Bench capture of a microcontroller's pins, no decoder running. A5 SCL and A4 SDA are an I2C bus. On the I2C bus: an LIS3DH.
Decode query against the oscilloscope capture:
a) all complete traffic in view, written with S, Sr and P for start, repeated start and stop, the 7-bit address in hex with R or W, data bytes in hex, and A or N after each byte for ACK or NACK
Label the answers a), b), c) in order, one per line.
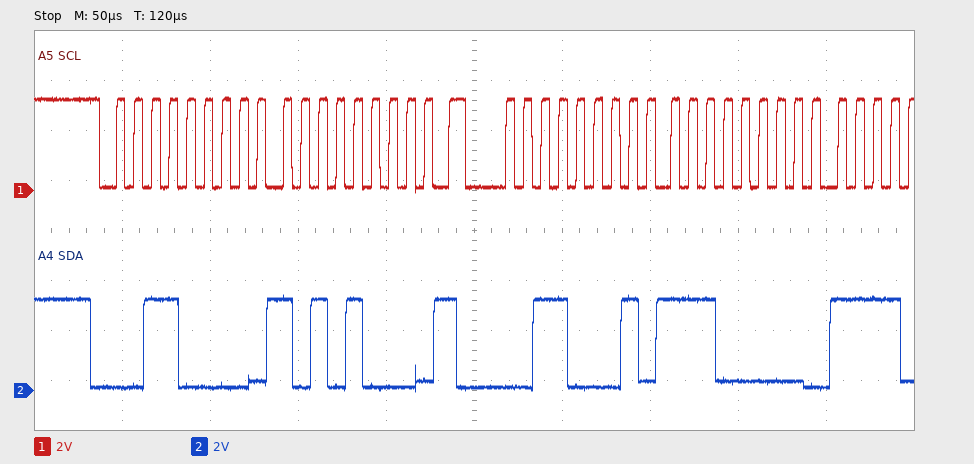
a) S 18W A A8 A Sr 18R A E0 A
